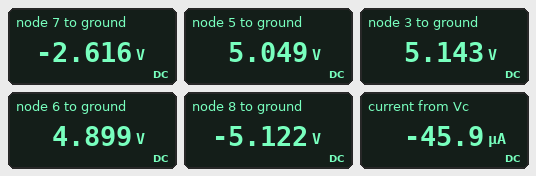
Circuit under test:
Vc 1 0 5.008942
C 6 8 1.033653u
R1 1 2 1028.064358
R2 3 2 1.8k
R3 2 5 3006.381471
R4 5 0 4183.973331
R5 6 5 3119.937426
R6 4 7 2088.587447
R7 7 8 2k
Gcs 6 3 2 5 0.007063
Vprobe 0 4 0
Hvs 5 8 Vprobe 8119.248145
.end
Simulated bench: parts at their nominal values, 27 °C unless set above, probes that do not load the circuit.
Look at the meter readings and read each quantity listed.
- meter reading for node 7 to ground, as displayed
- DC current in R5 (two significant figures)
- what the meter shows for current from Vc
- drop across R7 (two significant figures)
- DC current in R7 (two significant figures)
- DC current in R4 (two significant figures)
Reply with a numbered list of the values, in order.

1. -2.616 V
2. 48 µA
3. -45.9 µA
4. 2.5 V
5. 1.3 mA
6. 1.2 mA
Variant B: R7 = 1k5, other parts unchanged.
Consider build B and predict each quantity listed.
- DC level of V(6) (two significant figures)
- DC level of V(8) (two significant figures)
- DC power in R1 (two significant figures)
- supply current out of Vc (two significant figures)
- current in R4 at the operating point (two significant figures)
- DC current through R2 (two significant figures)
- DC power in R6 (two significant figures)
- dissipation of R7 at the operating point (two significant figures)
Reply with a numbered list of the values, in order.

1. 5.2 V
2. -3.9 V
3. 8.4 µW
4. 90 µA
5. 1.2 mA
6. 95 µA
7. 2.5 mW
8. 1.8 mW
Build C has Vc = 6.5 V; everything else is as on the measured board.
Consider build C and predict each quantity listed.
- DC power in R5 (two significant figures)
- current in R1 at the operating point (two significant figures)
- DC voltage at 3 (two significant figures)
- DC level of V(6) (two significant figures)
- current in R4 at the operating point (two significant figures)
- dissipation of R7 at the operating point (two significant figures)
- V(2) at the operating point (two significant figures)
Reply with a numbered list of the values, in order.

1. 12 µW
2. 60 µA
3. 6.7 V
4. 6.4 V
5. 1.6 mA
6. 5.3 mW
7. 6.6 V
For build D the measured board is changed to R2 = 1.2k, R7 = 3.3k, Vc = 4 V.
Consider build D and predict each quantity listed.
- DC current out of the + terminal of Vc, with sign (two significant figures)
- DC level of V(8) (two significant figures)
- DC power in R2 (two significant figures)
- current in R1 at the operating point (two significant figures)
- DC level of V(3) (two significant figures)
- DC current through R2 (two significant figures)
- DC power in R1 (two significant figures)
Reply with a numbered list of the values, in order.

1. -570 µA
2. -8.9 V
3. 430 µW
4. 570 µA
5. 5.3 V
6. 600 µA
7. 340 µW
